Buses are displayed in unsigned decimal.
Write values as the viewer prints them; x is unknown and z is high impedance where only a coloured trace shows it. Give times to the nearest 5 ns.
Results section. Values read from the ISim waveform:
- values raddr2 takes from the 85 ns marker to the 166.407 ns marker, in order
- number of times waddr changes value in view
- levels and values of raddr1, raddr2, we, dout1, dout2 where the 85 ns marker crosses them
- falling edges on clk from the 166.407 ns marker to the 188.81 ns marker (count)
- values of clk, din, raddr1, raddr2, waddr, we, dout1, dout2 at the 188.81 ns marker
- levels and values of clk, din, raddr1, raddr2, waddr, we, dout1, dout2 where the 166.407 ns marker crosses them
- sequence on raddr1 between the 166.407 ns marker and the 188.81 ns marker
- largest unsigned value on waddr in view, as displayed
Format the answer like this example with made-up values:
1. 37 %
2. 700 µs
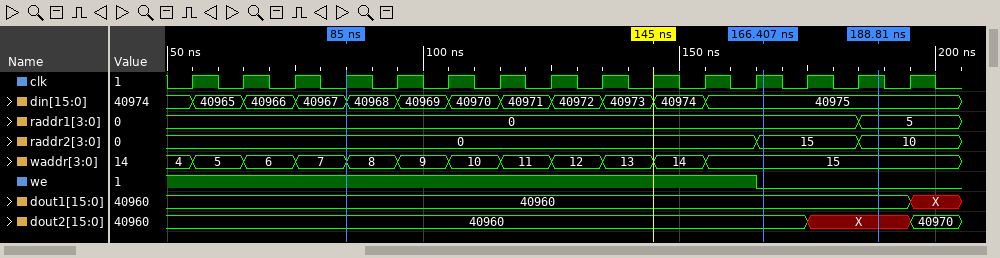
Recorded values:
1. 0, 15
2. 11
3. raddr1=0, raddr2=0, we=1, dout1=40960, dout2=40960
4. 2
5. clk=1, din=40975, raddr1=5, raddr2=10, waddr=15, we=0, dout1=40960, dout2=X
6. clk=1, din=40975, raddr1=0, raddr2=15, waddr=15, we=0, dout1=40960, dout2=40960
7. 0, 5
8. 15
